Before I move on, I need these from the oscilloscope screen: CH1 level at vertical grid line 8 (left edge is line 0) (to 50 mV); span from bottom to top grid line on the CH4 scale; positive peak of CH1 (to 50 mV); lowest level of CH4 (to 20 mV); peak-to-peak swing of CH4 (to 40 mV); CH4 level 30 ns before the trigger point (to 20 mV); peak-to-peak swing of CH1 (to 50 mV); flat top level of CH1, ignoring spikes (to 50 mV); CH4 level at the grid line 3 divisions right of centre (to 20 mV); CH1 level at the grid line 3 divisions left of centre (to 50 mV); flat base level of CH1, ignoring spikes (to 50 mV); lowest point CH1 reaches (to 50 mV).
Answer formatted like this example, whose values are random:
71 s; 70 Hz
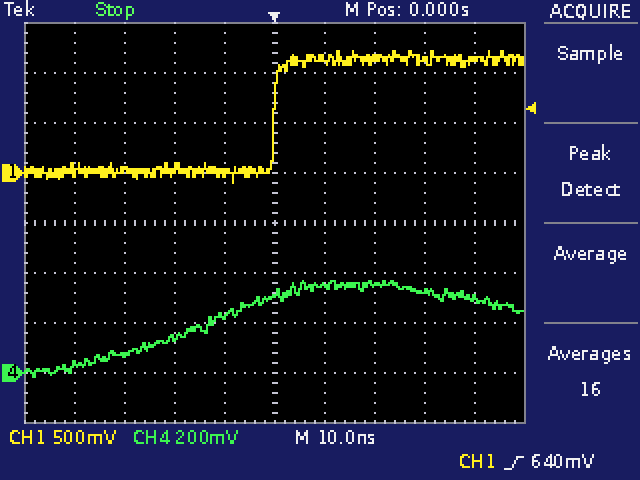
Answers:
1.10 V; 1.6 V; 1.20 V; -20 mV; 400 mV; 80 mV; 1.30 V; 1.15 V; 320 mV; 50 mV; 0 mV; -100 mV
